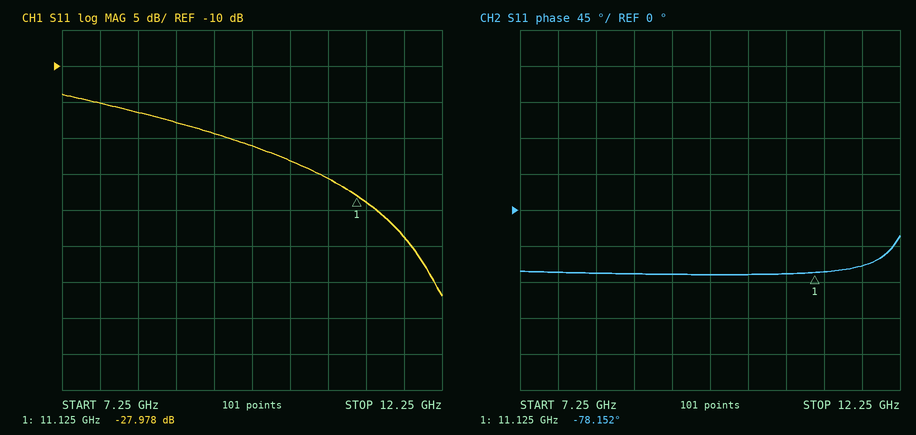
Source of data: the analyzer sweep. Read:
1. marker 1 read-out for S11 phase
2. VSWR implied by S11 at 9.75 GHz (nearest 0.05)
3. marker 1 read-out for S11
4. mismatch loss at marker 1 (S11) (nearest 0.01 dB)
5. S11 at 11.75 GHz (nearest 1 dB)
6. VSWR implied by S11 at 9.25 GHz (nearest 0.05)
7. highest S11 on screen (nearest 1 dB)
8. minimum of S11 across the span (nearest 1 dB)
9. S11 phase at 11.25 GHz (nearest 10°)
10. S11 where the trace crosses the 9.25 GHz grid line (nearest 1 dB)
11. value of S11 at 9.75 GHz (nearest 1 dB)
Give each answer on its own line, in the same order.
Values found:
-78.152°
1.20
-27.978 dB
0.01 dB
-34 dB
1.25
-14 dB
-42 dB
-80°
-19 dB
-21 dB
